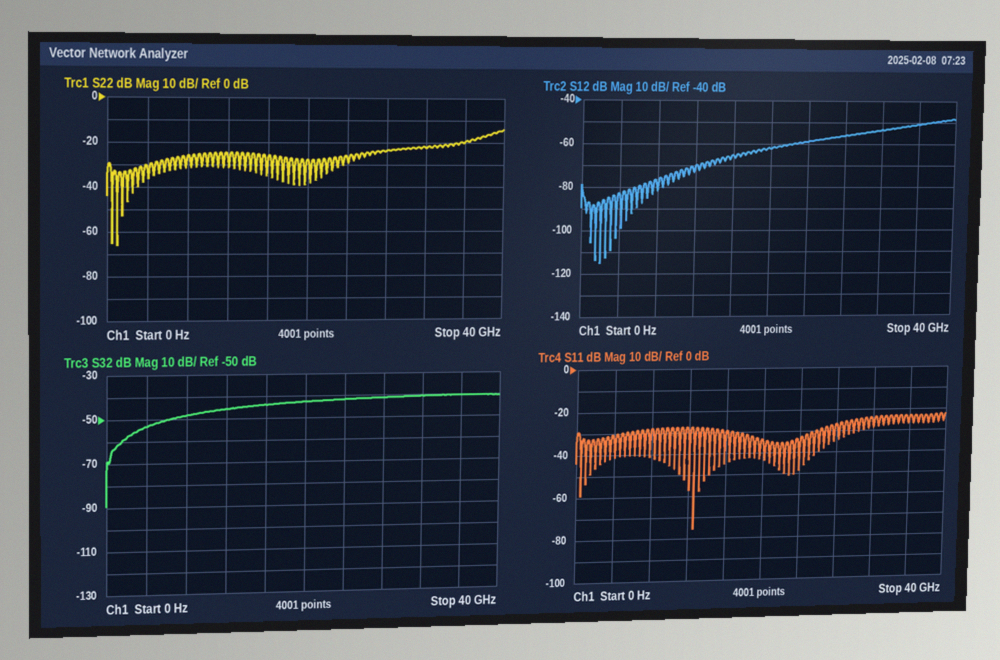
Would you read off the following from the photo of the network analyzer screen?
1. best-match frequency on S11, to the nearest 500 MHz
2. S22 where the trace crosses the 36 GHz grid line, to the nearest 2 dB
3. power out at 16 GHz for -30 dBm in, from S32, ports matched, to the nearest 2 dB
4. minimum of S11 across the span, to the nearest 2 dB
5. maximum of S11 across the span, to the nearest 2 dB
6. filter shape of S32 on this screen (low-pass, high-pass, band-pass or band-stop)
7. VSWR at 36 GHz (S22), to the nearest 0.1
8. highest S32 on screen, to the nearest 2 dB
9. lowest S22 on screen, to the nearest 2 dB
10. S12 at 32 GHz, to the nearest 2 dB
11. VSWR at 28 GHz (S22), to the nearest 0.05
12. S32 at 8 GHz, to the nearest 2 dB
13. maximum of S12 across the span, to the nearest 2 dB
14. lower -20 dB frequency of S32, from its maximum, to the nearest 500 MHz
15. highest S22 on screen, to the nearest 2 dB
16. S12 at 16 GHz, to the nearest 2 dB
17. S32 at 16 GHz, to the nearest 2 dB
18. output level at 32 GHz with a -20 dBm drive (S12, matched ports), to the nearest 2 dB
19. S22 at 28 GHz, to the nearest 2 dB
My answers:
12.5 GHz
-20 dB
-74 dBm
-76 dB
-22 dB
high-pass
1.2
-40 dB
-66 dB
-54 dB
1.15
-48 dB
-48 dB
1.5 GHz
-14 dB
-66 dB
-44 dB
-74 dBm
-24 dB
